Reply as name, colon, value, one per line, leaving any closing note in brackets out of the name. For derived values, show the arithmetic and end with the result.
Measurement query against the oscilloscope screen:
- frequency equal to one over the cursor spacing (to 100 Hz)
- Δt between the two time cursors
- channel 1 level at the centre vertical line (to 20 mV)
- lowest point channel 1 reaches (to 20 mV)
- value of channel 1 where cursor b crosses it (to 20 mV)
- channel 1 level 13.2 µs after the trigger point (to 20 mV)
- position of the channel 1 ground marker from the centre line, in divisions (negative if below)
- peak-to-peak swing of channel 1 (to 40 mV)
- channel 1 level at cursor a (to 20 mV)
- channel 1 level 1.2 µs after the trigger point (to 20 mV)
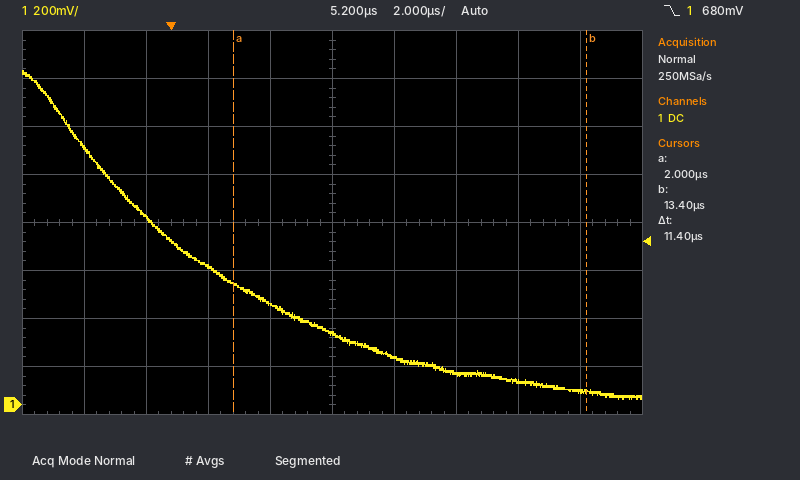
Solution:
frequency equal to one over the cursor spacing: 1 / 11.4 µs ≈ 87.7 kHz
Δt between the two time cursors: 11.4 µs
channel 1 level at the centre vertical line: 300 mV
lowest point channel 1 reaches: 20 mV
value of channel 1 where cursor b crosses it: 60 mV
channel 1 level 13.2 µs after the trigger point: 60 mV
position of the channel 1 ground marker from the centre line, in divisions: -3.8 div
peak-to-peak swing of channel 1: 1.36 V
channel 1 level at cursor a: 500 mV
channel 1 level 1.2 µs after the trigger point: 580 mV
